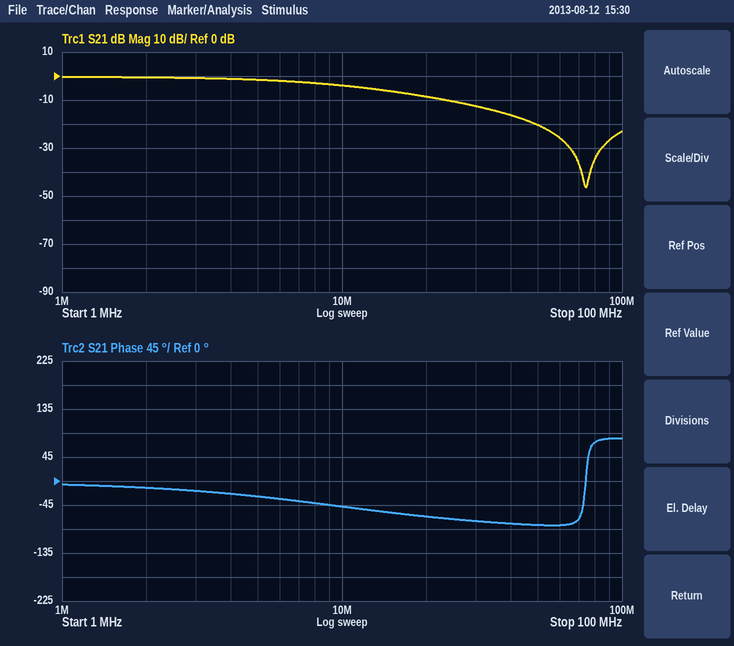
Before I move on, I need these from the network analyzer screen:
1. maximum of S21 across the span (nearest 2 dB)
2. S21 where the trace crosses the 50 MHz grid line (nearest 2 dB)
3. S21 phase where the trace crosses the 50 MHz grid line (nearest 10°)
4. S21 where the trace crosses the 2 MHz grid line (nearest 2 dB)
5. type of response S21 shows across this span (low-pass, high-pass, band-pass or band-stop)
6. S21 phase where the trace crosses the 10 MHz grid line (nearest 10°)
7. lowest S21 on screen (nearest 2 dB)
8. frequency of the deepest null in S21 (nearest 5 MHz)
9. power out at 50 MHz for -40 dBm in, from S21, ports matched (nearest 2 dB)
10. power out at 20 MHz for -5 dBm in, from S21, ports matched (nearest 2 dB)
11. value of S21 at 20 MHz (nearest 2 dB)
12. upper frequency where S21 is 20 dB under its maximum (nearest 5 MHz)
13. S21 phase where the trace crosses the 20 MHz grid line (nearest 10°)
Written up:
0 dB
-20 dB
-80°
0 dB
low-pass
-50°
-46 dB
75 MHz
-60 dBm
-14 dBm
-8 dB
50 MHz
-70°
